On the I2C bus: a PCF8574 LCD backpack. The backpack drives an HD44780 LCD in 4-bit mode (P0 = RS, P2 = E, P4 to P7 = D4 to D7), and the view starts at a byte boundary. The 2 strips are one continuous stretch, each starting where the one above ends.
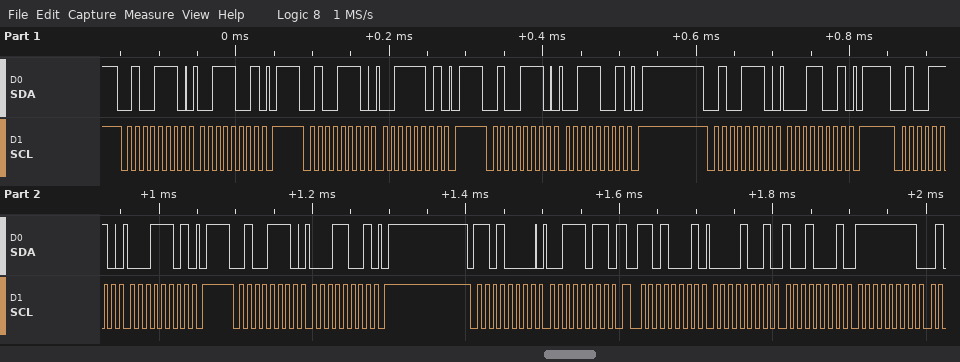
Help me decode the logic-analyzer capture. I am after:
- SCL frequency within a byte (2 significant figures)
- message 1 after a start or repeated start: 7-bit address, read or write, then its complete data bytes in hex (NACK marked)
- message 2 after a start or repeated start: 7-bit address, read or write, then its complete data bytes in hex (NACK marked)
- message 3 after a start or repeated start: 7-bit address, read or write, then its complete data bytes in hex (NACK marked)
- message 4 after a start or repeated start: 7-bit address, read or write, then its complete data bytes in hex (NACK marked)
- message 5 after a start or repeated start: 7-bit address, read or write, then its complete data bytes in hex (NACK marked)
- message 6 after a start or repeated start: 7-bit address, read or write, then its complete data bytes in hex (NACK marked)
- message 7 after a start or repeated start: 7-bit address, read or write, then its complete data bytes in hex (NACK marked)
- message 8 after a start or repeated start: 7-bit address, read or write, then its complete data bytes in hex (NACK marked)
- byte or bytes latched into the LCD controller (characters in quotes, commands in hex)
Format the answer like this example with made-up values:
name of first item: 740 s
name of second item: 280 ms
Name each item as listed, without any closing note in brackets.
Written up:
SCL frequency within a byte: 100 kHz
message 1 after a start or repeated start: 7-bit address, read or write, then its complete data bytes in hex: 0x27 write: 39
message 2 after a start or repeated start: 7-bit address, read or write, then its complete data bytes in hex: 0x27 write: 3D
message 3 after a start or repeated start: 7-bit address, read or write, then its complete data bytes in hex: 0x27 write: 39
message 4 after a start or repeated start: 7-bit address, read or write, then its complete data bytes in hex: 0x27 write: 19
message 5 after a start or repeated start: 7-bit address, read or write, then its complete data bytes in hex: 0x27 write: 1D
message 6 after a start or repeated start: 7-bit address, read or write, then its complete data bytes in hex: 0x27 write: 19
message 7 after a start or repeated start: 7-bit address, read or write, then its complete data bytes in hex: 0x68 write: 3B
message 8 after a start or repeated start: 7-bit address, read or write, then its complete data bytes in hex: 0x68 read: 09 91 FF
byte or bytes latched into the LCD controller: '1'
